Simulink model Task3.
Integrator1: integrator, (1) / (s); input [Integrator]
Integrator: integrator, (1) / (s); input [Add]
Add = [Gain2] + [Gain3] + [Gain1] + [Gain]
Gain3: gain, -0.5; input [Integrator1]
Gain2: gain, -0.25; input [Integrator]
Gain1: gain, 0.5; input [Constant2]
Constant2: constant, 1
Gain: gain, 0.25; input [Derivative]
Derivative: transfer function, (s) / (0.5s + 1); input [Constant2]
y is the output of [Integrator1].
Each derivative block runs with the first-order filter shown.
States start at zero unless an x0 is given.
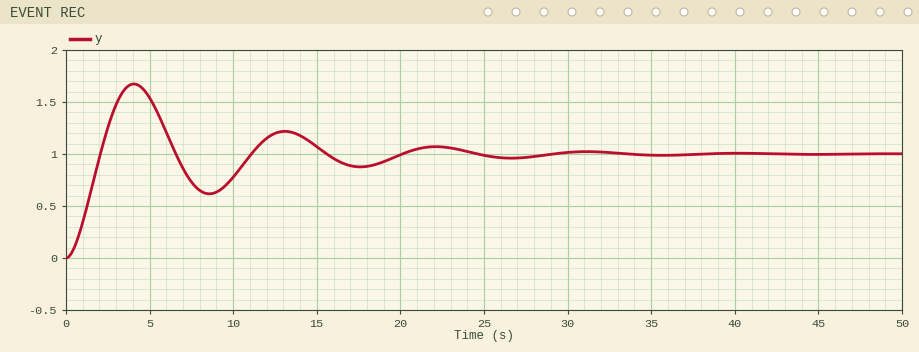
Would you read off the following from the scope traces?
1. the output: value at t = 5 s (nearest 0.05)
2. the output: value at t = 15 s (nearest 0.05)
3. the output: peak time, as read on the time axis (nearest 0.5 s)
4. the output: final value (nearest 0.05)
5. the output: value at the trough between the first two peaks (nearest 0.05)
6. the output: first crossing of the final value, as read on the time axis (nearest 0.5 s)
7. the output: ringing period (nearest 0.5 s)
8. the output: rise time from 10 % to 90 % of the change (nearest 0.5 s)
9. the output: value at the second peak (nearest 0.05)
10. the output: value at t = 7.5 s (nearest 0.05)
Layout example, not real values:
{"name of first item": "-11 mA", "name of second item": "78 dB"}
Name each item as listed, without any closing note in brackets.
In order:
{"the output: value at t = 5 s": "1.55", "the output: value at t = 15 s": "1.05", "the output: peak time, as read on the time axis": "4.0 s", "the output: final value": "1.00", "the output: value at the trough between the first two peaks": "0.60", "the output: first crossing of the final value, as read on the time axis": "2.0 s", "the output: ringing period": "9.0 s", "the output: rise time from 10 % to 90 % of the change": "1.5 s", "the output: value at the second peak": "1.20", "the output: value at t = 7.5 s": "0.75"}
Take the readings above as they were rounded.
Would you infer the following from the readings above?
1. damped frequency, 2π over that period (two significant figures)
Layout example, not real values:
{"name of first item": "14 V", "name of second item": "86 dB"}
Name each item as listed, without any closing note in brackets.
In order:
{"damped frequency, 2π over that period": "0.70 rad/s"}
